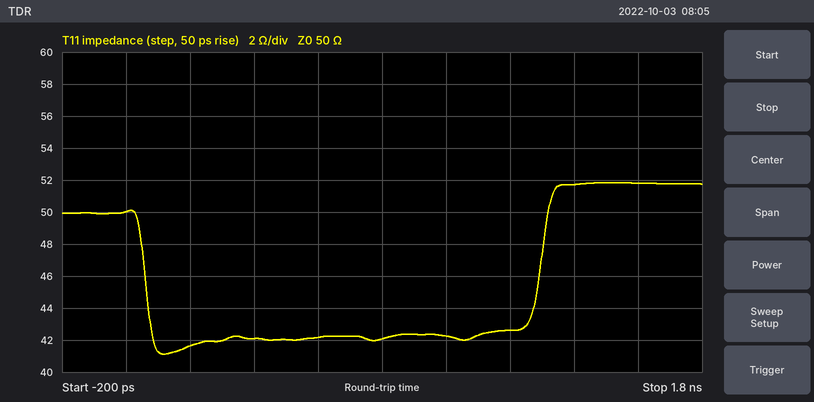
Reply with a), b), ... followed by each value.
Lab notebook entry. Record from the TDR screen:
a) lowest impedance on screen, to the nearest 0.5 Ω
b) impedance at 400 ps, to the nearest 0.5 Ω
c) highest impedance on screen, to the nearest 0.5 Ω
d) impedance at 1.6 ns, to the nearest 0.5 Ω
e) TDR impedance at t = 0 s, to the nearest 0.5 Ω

a) 41.0 Ω
b) 42.0 Ω
c) 52.0 Ω
d) 52.0 Ω
e) 50.0 Ω
